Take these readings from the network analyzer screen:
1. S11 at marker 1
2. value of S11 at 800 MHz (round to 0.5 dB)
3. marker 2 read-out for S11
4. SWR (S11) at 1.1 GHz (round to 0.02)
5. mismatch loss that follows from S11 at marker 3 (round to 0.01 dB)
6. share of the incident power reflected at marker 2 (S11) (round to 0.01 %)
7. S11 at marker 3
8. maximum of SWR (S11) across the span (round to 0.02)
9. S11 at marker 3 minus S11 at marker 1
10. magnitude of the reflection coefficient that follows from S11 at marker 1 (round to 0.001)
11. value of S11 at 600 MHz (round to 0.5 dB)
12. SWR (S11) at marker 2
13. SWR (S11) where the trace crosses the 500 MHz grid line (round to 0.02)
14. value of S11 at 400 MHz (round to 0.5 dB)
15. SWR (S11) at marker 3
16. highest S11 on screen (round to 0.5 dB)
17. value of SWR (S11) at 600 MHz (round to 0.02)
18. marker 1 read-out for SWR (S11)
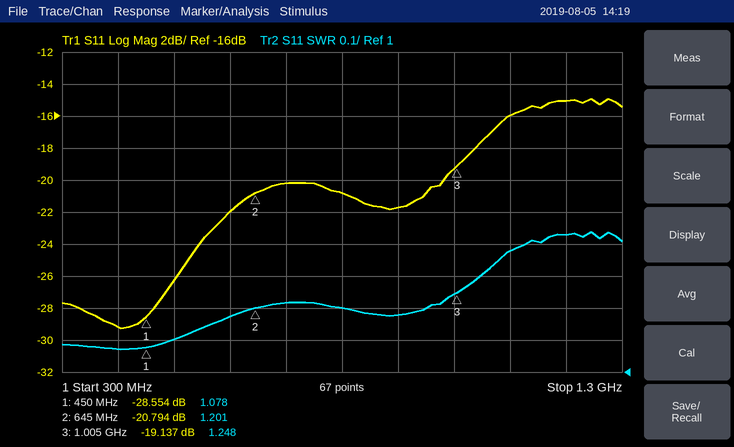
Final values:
-28.554 dB
-21.0 dB
-20.794 dB
1.38
0.05 dB
0.83 %
-19.137 dB
1.44
9.417 dB
0.037
-22.0 dB
1.201
1.10
-29.0 dB
1.248
-15.0 dB
1.18
1.078
